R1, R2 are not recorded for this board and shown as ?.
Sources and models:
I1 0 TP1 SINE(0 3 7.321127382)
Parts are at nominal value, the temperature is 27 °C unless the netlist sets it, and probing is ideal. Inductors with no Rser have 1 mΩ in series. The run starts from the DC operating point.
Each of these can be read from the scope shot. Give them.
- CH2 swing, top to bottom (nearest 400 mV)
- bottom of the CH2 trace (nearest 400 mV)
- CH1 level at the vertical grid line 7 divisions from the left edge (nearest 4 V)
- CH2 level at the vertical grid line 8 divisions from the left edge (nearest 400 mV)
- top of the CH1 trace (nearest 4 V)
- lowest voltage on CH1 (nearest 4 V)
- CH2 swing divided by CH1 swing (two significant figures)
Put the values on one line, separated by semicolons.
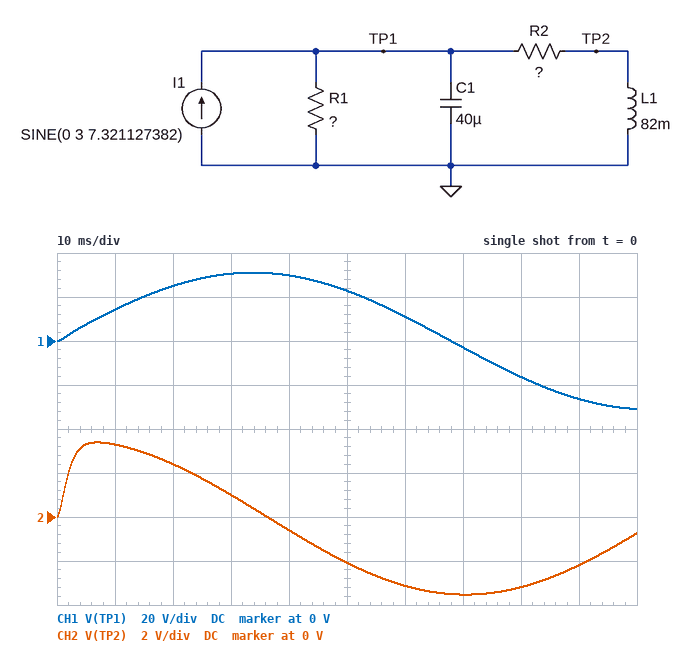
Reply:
6.8 V; -3.6 V; -4 V; -3.2 V; 32 V; -32 V; 0.11
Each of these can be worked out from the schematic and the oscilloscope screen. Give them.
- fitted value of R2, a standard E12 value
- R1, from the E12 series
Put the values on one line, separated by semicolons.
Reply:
33 Ω; 15 Ω
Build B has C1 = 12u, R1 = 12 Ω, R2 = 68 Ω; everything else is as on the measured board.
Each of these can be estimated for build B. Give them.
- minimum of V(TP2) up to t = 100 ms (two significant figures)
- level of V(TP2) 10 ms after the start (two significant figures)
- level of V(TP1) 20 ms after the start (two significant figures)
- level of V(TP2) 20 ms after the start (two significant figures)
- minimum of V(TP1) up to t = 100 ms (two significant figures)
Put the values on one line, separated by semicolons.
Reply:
-1.7 V; 1.6 V; 24 V; 1.1 V; -30 V
